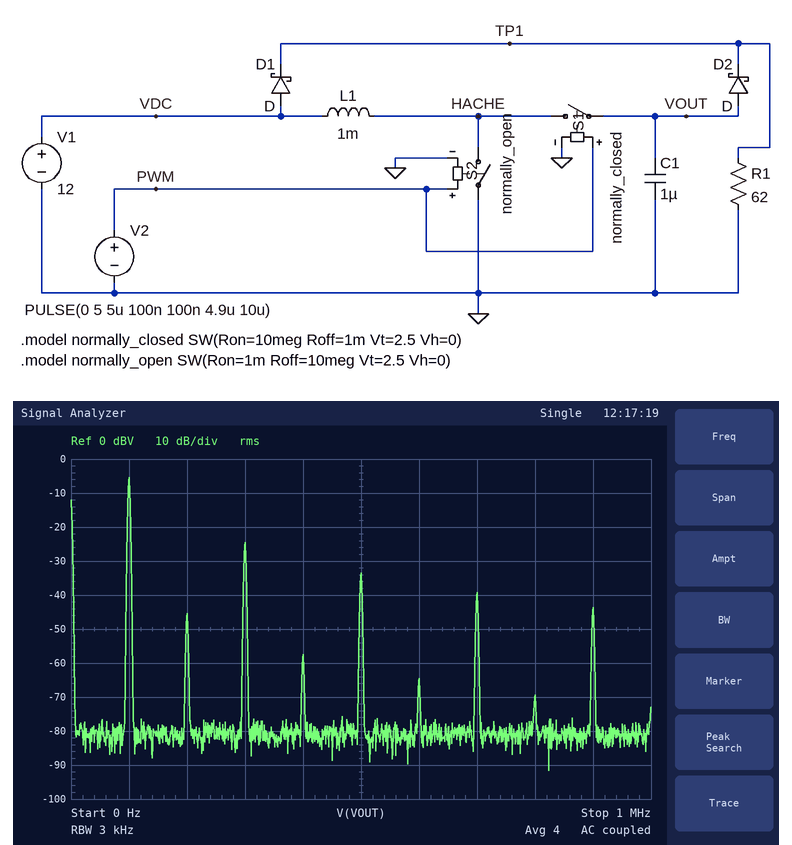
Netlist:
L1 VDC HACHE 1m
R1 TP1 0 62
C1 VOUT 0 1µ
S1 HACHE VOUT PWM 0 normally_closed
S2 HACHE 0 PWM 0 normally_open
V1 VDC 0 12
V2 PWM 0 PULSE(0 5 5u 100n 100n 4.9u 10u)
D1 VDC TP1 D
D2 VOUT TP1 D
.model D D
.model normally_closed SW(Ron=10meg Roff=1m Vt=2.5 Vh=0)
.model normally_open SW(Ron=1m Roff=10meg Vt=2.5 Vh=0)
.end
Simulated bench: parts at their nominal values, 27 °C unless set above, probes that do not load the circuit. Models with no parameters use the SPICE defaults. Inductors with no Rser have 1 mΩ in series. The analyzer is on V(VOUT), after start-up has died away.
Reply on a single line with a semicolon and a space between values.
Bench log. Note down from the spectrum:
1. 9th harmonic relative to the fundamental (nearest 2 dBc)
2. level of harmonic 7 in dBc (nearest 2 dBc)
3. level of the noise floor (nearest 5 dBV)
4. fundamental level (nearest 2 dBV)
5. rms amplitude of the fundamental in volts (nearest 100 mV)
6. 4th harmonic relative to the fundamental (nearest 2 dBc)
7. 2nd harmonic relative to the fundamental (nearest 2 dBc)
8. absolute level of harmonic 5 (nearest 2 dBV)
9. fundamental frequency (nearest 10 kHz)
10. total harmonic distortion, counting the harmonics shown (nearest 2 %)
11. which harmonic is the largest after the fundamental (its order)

-38 dBc; -34 dBc; -80 dBV; -6 dBV; 500 mV; -52 dBc; -40 dBc; -34 dBV; 100 kHz; 12 %; 3
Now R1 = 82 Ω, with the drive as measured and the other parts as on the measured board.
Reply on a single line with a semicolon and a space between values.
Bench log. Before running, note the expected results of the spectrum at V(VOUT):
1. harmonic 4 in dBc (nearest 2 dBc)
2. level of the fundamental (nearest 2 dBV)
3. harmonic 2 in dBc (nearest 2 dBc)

-50 dBc; -8 dBV; -38 dBc
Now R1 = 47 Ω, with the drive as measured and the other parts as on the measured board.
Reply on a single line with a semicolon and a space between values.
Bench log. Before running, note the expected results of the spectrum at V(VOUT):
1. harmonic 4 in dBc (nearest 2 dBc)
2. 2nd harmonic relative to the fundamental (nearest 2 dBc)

-54 dBc; -42 dBc
